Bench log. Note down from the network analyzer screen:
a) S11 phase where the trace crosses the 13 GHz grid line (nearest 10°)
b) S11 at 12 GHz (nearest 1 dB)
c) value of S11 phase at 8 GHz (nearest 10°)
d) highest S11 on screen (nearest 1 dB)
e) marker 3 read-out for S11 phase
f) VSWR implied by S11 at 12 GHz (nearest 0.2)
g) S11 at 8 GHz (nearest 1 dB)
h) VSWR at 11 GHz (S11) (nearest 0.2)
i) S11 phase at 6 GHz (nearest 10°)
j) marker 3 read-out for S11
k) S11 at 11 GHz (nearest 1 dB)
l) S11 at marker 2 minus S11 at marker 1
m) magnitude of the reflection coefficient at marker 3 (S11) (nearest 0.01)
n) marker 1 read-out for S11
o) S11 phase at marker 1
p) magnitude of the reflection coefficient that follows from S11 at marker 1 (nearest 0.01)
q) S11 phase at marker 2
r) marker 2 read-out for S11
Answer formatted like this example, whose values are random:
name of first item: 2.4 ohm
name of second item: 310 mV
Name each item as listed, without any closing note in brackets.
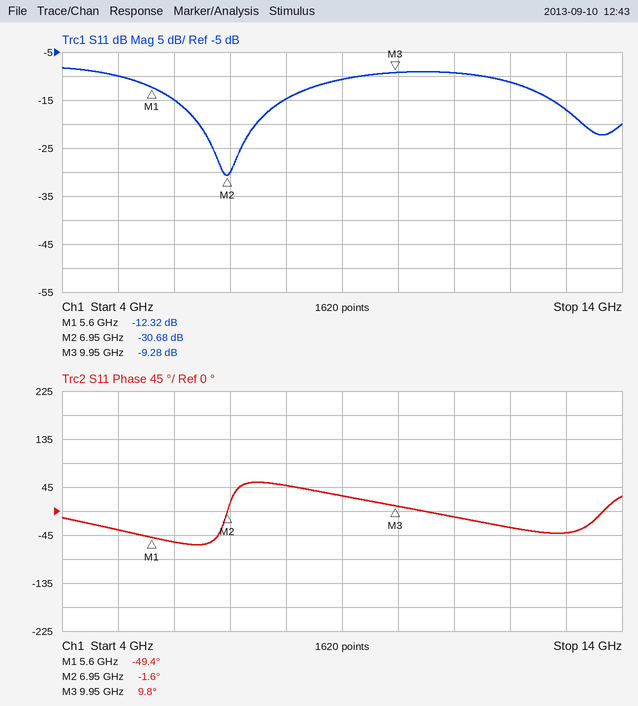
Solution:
S11 phase where the trace crosses the 13 GHz grid line: -40°
S11 at 12 GHz: -11 dB
value of S11 phase at 8 GHz: 50°
highest S11 on screen: -8 dB
marker 3 read-out for S11 phase: 9.8°
VSWR implied by S11 at 12 GHz: 1.8
S11 at 8 GHz: -15 dB
VSWR at 11 GHz (S11): 2.0
S11 phase at 6 GHz: -60°
marker 3 read-out for S11: -9.28 dB
S11 at 11 GHz: -9 dB
S11 at marker 2 minus S11 at marker 1: -18.36 dB
magnitude of the reflection coefficient at marker 3 (S11): 0.34
marker 1 read-out for S11: -12.32 dB
S11 phase at marker 1: -49.4°
magnitude of the reflection coefficient that follows from S11 at marker 1: 0.24
S11 phase at marker 2: -1.6°
marker 2 read-out for S11: -30.68 dB
